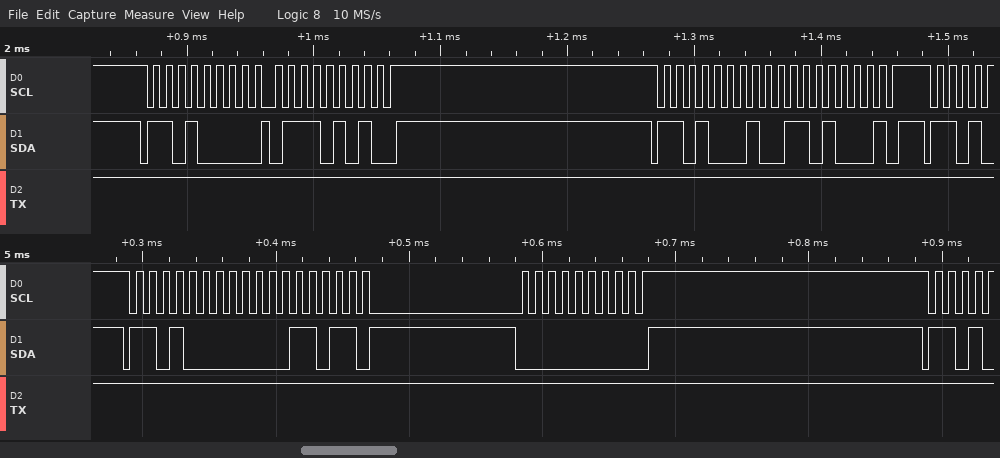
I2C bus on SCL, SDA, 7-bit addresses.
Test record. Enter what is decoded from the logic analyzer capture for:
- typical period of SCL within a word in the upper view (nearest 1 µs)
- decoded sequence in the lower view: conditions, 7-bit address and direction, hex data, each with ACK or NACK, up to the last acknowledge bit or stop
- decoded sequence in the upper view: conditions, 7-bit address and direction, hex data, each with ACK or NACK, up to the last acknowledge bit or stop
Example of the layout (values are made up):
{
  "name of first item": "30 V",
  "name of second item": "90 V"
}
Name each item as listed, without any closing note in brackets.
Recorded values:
{
  "typical period of SCL within a word in the upper view": "10 µs",
  "decoded sequence in the lower view: conditions, 7-bit address and direction, hex data, each with ACK or NACK, up to the last acknowledge bit or stop": "start, address 68 write ACK, 1B ACK, 00 ACK, stop",
  "decoded sequence in the upper view: conditions, 7-bit address and direction, hex data, each with ACK or NACK, up to the last acknowledge bit or stop": "start, address 68 write ACK, 75 ACK, stop, start, address 68 read ACK, 68 NACK, stop"
}
